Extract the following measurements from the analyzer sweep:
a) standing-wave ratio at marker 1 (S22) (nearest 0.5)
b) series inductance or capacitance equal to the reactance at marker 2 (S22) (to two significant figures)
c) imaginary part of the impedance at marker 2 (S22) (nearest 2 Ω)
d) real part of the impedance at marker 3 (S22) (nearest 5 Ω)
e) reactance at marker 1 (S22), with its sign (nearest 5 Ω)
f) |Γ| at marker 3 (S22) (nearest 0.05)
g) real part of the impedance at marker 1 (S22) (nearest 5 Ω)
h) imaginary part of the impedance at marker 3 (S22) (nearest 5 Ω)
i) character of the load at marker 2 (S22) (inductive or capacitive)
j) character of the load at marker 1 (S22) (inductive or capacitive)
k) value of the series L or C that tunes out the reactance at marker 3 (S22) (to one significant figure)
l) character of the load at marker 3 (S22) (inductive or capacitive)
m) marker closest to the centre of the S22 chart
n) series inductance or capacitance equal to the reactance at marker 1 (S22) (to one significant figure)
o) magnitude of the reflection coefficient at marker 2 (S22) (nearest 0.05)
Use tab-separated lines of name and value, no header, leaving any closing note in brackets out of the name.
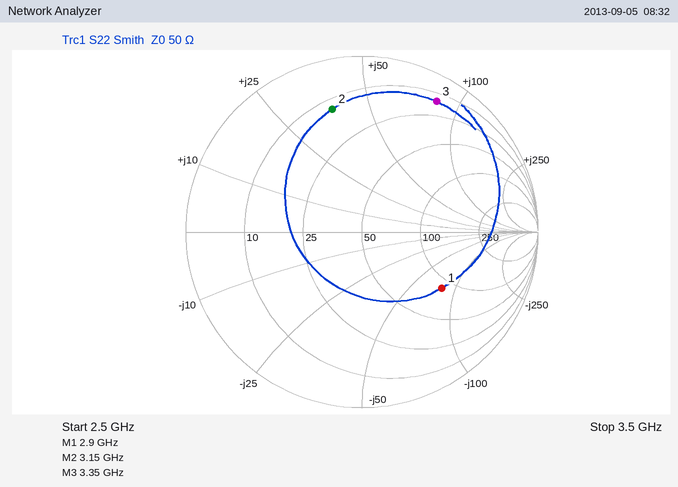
standing-wave ratio at marker 1 (S22)	3.5
series inductance or capacitance equal to the reactance at marker 2 (S22)	1.9 nH
imaginary part of the impedance at marker 2 (S22)	+38 Ω
real part of the impedance at marker 3 (S22)	15 Ω
reactance at marker 1 (S22), with its sign	-80 Ω
|Γ| at marker 3 (S22)	0.85
real part of the impedance at marker 1 (S22)	85 Ω
imaginary part of the impedance at marker 3 (S22)	+85 Ω
character of the load at marker 2 (S22)	inductive
character of the load at marker 1 (S22)	capacitive
value of the series L or C that tunes out the reactance at marker 3 (S22)	600 fF
character of the load at marker 3 (S22)	inductive
marker closest to the centre of the S22 chart	marker 1
series inductance or capacitance equal to the reactance at marker 1 (S22)	700 fF
magnitude of the reflection coefficient at marker 2 (S22)	0.70
